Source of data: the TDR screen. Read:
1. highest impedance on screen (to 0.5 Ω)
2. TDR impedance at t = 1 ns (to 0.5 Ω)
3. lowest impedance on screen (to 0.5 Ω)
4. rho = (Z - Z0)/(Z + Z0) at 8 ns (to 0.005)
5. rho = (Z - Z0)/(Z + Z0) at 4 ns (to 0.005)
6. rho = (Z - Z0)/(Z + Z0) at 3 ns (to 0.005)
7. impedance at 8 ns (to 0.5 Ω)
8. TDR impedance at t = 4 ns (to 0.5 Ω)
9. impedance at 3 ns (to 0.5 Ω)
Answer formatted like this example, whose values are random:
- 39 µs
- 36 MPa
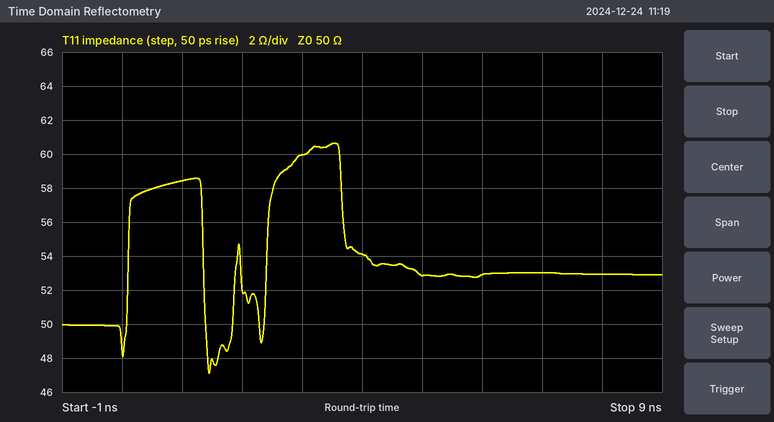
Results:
- 60.5 Ω
- 58.5 Ω
- 47.0 Ω
- +0.030
- +0.040
- +0.090
- 53.0 Ω
- 54.0 Ω
- 60.0 Ω
